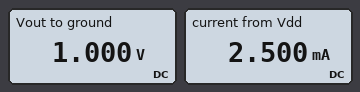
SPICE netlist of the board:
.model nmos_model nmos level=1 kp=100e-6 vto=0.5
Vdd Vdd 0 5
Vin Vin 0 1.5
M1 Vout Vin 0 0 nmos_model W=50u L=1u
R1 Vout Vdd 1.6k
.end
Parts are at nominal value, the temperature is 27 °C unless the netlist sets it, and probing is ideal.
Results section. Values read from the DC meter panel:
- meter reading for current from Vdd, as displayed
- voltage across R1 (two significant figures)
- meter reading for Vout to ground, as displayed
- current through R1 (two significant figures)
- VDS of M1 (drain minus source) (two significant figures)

2.500 mA
4.0 V
1.000 V
2.5 mA
1.0 V
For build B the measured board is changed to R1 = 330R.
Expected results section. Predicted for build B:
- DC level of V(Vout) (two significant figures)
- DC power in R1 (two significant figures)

4.2 V
2.1 mW
